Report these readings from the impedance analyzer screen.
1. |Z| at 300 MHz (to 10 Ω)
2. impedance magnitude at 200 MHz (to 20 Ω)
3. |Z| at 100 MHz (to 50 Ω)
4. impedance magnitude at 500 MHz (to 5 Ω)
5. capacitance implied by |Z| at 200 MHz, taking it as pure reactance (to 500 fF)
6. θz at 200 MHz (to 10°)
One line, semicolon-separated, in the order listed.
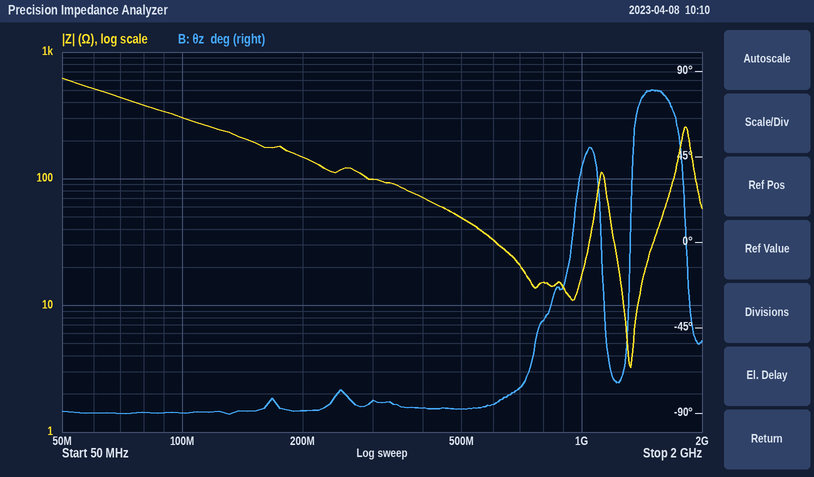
100 Ω; 140 Ω; 300 Ω; 50 Ω; 5.5 pF; -90°
